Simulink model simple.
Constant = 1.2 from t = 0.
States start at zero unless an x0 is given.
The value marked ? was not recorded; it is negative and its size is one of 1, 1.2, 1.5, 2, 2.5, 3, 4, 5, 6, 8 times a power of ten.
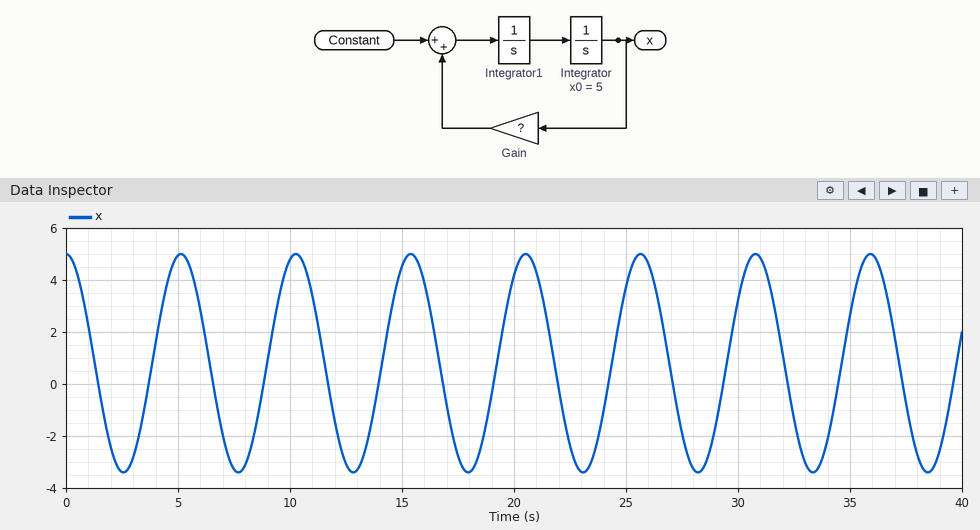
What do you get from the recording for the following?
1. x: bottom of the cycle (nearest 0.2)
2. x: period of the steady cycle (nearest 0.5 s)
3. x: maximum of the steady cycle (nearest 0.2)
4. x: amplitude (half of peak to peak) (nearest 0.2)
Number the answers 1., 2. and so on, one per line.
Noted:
1. -3.4
2. 5.0 s
3. 5.0
4. 4.2
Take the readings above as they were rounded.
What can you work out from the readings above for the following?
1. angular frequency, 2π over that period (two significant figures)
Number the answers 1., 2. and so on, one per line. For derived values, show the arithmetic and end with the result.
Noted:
1. 2π / 5 = 1.3 rad/s
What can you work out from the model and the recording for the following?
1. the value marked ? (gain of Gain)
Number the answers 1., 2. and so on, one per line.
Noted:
1. -1.5
